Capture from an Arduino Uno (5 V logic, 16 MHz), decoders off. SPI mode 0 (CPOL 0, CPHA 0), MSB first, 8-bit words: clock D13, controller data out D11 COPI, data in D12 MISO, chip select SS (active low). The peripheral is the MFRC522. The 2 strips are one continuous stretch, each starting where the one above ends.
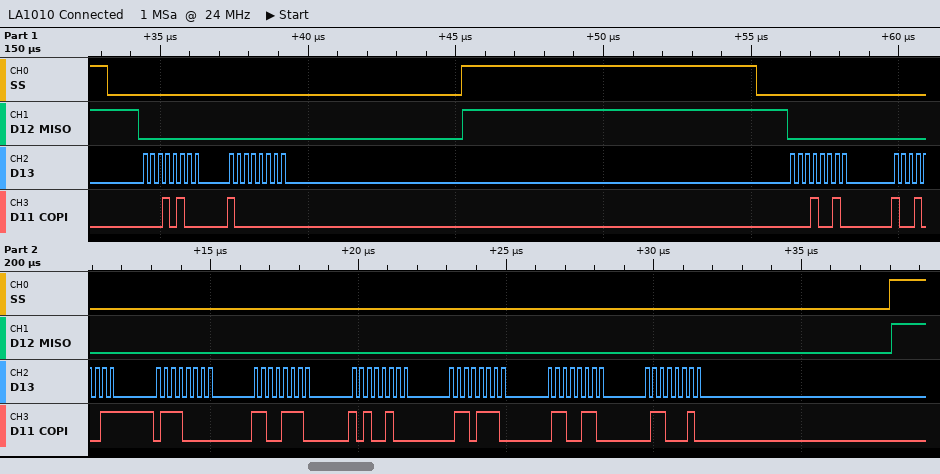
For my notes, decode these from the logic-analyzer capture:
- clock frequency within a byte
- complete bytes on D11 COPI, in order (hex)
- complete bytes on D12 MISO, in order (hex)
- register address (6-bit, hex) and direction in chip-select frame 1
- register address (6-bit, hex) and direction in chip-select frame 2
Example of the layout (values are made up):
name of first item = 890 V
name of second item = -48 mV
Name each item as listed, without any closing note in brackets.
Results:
clock frequency within a byte = 4 MHz
complete bytes on D11 COPI, in order = 0x14 0x80 0x12 0x93 0x70 0xCE 0xA4 0x6E 0x66 0x62
complete bytes on D12 MISO, in order = 0x00 0x00 0x00 0x00 0x00 0x00 0x00 0x00 0x00 0x00
register address (6-bit, hex) and direction in chip-select frame 1 = 0x0A write
register address (6-bit, hex) and direction in chip-select frame 2 = 0x09 write
